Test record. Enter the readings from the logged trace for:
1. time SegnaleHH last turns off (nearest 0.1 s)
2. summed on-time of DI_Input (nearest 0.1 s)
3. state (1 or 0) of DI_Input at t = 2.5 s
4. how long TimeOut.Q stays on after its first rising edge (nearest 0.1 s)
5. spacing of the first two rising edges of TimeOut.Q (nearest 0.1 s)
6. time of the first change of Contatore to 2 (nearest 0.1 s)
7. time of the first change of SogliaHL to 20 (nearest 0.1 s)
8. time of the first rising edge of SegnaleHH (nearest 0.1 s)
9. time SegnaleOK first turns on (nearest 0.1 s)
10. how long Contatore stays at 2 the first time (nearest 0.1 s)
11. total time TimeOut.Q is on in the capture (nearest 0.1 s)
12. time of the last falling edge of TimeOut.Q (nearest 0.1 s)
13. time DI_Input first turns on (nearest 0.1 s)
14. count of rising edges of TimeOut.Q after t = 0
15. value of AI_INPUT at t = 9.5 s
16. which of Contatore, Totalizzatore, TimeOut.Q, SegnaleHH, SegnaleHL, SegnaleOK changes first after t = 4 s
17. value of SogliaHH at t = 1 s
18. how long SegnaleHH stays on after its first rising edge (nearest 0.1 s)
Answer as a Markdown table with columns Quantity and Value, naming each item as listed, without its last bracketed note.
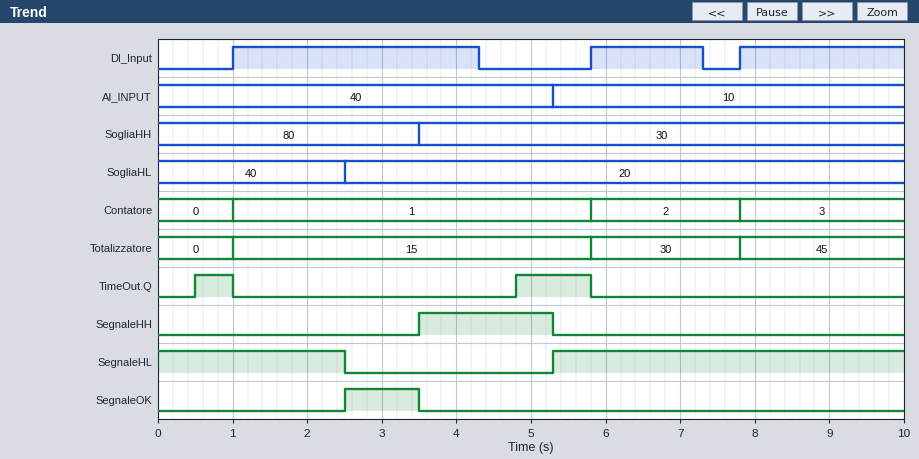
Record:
| Quantity | Value |
|---|---|
| time SegnaleHH last turns off | 5.3 s |
| summed on-time of DI_Input | 7.0 s |
| state (1 or 0) of DI_Input at t = 2.5 s | 1 |
| how long TimeOut.Q stays on after its first rising edge | 0.5 s |
| spacing of the first two rising edges of TimeOut.Q | 4.3 s |
| time of the first change of Contatore to 2 | 5.8 s |
| time of the first change of SogliaHL to 20 | 2.5 s |
| time of the first rising edge of SegnaleHH | 3.5 s |
| time SegnaleOK first turns on | 2.5 s |
| how long Contatore stays at 2 the first time | 2.0 s |
| total time TimeOut.Q is on in the capture | 1.5 s |
| time of the last falling edge of TimeOut.Q | 5.8 s |
| time DI_Input first turns on | 1.0 s |
| count of rising edges of TimeOut.Q after t = 0 | 2 |
| value of AI_INPUT at t = 9.5 s | 10 |
| which of Contatore, Totalizzatore, TimeOut.Q, SegnaleHH, SegnaleHL, SegnaleOK changes first after t = 4 s | TimeOut.Q |
| value of SogliaHH at t = 1 s | 80 |
| how long SegnaleHH stays on after its first rising edge | 1.8 s |
